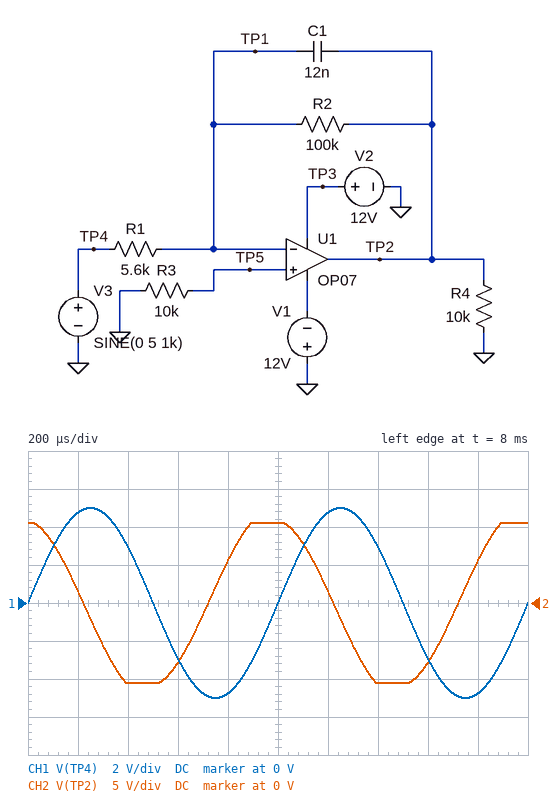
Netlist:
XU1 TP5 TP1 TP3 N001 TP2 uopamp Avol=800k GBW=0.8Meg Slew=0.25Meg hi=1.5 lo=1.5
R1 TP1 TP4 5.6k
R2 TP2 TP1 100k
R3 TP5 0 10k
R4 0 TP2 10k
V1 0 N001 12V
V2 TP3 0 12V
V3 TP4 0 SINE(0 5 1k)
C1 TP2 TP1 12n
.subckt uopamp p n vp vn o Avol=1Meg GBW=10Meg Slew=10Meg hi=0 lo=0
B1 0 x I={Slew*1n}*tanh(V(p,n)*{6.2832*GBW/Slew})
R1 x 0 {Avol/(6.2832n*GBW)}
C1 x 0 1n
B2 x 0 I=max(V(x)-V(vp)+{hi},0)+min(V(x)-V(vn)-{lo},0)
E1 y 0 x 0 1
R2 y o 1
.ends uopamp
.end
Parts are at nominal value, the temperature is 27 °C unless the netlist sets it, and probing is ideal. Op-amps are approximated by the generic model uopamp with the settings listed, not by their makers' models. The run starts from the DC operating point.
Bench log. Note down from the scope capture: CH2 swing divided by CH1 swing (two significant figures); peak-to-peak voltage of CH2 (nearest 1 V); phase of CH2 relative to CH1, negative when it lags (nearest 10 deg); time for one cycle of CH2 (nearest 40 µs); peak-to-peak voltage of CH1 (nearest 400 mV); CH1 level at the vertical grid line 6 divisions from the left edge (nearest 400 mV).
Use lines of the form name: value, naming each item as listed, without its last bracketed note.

CH2 swing divided by CH1 swing: 2.1
peak-to-peak voltage of CH2: 21 V
phase of CH2 relative to CH1, negative when it lags: 100 deg
time for one cycle of CH2: 1.00 ms
peak-to-peak voltage of CH1: 10.0 V
CH1 level at the vertical grid line 6 divisions from the left edge: 4.8 V
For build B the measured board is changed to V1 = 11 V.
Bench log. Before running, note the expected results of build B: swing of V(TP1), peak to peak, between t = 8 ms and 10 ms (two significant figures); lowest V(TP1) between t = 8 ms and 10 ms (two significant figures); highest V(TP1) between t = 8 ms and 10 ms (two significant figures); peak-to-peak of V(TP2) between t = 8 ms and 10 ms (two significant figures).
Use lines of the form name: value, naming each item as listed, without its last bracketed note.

swing of V(TP1), peak to peak, between t = 8 ms and 10 ms: 2.5 V
lowest V(TP1) between t = 8 ms and 10 ms: -1.2 V
highest V(TP1) between t = 8 ms and 10 ms: 1.3 V
peak-to-peak of V(TP2) between t = 8 ms and 10 ms: 20 V
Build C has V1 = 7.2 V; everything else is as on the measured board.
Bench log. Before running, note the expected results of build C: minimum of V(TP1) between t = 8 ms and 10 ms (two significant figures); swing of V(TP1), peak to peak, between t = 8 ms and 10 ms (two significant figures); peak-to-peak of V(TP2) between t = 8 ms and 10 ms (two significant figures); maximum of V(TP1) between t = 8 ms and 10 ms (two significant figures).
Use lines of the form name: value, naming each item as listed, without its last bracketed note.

minimum of V(TP1) between t = 8 ms and 10 ms: -2.0 V
swing of V(TP1), peak to peak, between t = 8 ms and 10 ms: 4.5 V
peak-to-peak of V(TP2) between t = 8 ms and 10 ms: 16 V
maximum of V(TP1) between t = 8 ms and 10 ms: 2.5 V
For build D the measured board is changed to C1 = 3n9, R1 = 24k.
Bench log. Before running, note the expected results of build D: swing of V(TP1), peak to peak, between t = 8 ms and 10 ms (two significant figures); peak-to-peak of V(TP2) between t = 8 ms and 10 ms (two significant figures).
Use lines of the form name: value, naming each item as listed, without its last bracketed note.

swing of V(TP1), peak to peak, between t = 8 ms and 10 ms: 20 mV
peak-to-peak of V(TP2) between t = 8 ms and 10 ms: 16 V
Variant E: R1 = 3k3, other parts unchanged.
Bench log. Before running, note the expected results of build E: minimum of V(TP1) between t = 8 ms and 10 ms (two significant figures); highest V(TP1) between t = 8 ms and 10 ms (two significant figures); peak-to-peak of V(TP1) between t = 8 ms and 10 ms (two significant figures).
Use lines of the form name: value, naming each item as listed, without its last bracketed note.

minimum of V(TP1) between t = 8 ms and 10 ms: -3.6 V
highest V(TP1) between t = 8 ms and 10 ms: 3.6 V
peak-to-peak of V(TP1) between t = 8 ms and 10 ms: 7.3 V
